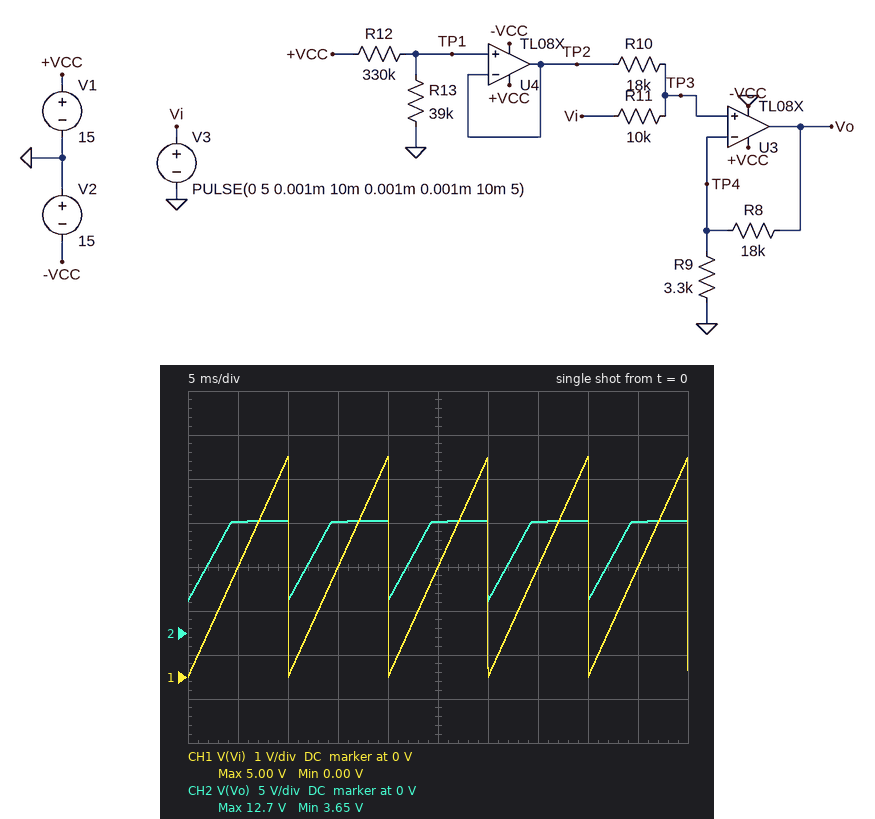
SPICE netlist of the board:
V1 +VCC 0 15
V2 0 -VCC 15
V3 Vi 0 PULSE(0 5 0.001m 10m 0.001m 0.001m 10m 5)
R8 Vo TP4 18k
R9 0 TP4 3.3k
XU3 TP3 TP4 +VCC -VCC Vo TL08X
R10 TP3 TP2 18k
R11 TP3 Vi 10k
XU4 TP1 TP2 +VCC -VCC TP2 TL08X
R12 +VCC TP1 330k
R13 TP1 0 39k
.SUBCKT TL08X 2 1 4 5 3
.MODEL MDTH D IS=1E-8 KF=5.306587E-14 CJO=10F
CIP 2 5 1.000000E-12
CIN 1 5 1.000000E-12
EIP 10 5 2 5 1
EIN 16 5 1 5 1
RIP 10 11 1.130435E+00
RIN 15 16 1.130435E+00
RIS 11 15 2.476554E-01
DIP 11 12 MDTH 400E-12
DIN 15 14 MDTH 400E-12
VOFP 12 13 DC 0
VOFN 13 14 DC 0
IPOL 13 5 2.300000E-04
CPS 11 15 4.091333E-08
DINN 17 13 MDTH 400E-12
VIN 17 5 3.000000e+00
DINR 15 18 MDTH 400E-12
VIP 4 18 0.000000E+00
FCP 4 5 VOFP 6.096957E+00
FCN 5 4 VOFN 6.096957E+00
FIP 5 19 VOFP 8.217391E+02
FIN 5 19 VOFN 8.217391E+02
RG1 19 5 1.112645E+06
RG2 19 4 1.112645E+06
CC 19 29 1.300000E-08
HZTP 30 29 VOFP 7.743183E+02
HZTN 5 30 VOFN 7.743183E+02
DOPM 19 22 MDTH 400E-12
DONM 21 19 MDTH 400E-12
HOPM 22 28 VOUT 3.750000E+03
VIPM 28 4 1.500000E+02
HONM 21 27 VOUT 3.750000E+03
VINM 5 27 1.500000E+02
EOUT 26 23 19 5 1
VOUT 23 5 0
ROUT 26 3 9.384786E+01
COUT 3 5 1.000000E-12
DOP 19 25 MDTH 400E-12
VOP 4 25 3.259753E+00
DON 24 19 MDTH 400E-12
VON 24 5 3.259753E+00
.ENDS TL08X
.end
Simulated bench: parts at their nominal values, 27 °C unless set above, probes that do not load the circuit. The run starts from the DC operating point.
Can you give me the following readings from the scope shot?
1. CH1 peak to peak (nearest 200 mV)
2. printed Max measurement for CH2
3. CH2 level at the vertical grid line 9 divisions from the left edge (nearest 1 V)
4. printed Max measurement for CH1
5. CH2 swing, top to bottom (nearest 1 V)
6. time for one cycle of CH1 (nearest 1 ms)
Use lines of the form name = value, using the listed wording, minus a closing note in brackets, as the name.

CH1 peak to peak = 5.0 V
printed Max measurement for CH2 = 12.7 V
CH2 level at the vertical grid line 9 divisions from the left edge = 13 V
printed Max measurement for CH1 = 5.00 V
CH2 swing, top to bottom = 9 V
time for one cycle of CH1 = 10 ms
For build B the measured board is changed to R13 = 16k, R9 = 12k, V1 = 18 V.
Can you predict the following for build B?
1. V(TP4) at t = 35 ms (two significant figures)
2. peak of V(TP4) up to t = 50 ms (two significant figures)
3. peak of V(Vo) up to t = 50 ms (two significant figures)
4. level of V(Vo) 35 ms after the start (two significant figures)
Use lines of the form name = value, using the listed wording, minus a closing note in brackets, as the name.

V(TP4) at t = 35 ms = 1.9 V
peak of V(TP4) up to t = 50 ms = 3.5 V
peak of V(Vo) up to t = 50 ms = 8.9 V
level of V(Vo) 35 ms after the start = 4.8 V
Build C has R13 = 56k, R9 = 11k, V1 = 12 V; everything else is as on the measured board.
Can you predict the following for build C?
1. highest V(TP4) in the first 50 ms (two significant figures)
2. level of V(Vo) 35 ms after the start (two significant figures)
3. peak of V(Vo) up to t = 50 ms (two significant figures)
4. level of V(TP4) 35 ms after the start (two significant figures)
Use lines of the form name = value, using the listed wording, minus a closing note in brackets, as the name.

highest V(TP4) in the first 50 ms = 3.7 V
level of V(Vo) 35 ms after the start = 5.9 V
peak of V(Vo) up to t = 50 ms = 9.7 V
level of V(TP4) 35 ms after the start = 2.2 V
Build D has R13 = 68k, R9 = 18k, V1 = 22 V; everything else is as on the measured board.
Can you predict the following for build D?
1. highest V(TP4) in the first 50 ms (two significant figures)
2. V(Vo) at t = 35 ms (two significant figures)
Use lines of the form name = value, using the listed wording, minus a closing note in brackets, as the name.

highest V(TP4) in the first 50 ms = 4.6 V
V(Vo) at t = 35 ms = 5.9 V
